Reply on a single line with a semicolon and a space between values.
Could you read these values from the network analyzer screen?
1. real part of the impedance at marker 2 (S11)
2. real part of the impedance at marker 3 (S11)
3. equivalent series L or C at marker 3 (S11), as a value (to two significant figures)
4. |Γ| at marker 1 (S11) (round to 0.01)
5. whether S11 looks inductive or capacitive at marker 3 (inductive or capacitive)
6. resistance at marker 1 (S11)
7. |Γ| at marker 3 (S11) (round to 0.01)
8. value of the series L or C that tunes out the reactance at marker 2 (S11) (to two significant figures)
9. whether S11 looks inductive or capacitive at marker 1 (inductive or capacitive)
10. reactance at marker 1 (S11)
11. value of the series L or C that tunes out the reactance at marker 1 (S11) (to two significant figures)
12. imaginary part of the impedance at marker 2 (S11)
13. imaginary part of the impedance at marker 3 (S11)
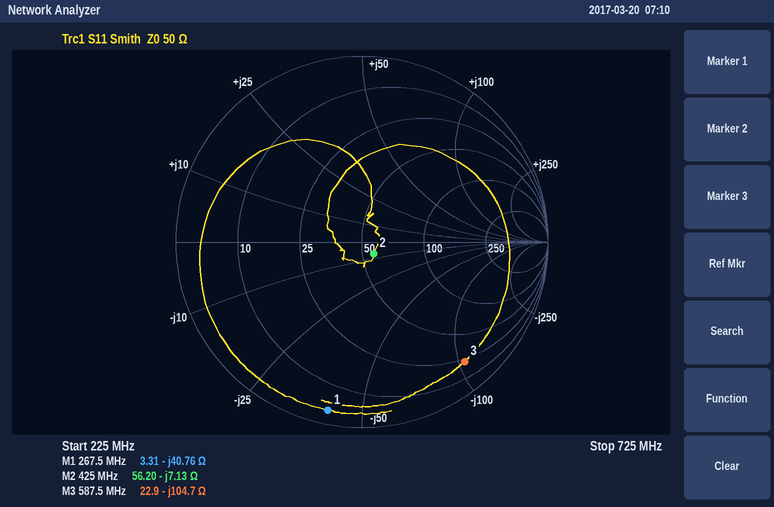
56.20 Ω; 22.9 Ω; 2.6 pF; 0.92; capacitive; 3.31 Ω; 0.85; 2.7 nH; capacitive; -40.76 Ω; 24 nH; -7.13 Ω; -104.7 Ω
